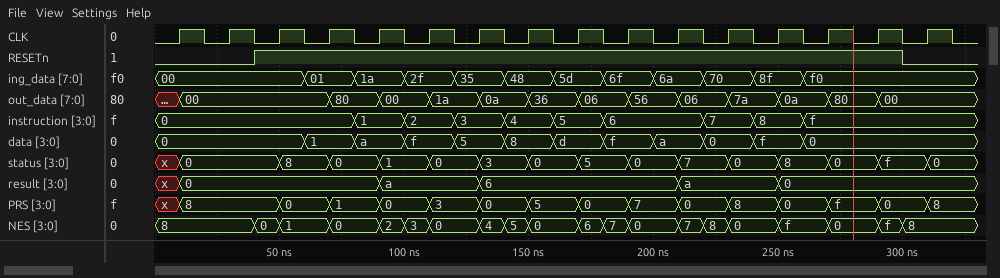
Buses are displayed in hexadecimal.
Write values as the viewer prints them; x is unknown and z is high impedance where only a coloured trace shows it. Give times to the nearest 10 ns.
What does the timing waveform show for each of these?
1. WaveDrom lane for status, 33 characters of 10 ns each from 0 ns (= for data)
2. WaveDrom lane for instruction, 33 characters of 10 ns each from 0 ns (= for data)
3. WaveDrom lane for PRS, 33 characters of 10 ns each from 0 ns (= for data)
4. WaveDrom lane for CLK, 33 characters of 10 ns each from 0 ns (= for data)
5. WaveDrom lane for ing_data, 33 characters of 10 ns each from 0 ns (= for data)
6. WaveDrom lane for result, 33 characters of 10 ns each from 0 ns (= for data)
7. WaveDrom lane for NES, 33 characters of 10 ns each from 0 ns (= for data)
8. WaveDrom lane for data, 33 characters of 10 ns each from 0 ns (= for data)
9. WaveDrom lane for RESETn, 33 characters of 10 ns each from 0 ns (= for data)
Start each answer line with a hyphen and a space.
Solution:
- {name: 'status', wave: 'x=...=.=.=.=.=.=.=.=.=.=.=.=.=.=.', data: '0 8 0 1 0 3 0 5 0 7 0 8 0 f 0'}
- {name: 'instruction', wave: '=.......=.=.=.=.=.=...=.=.=......', data: '0 1 2 3 4 5 6 7 8 f'}
- {name: 'PRS', wave: 'x=...=.=.=.=.=.=.=.=.=.=.=.=.=.=.', data: '8 0 1 0 3 0 5 0 7 0 8 0 f 0 8'}
- {name: 'CLK', wave: '010101010101010101010101010101010'}
- {name: 'ing_data', wave: '=.....=.=.=.=.=.=.=.=.=.=.=......', data: '00 01 1a 2f 35 48 5d 6f 6a 70 8f f0'}
- {name: 'result', wave: 'x=.......=...=.......=...=.......', data: '0 a 6 a 0'}
- {name: 'NES', wave: '=...==.=.===.===.===.===.=.=.==..', data: '8 0 1 0 2 3 0 4 5 0 6 7 0 7 8 0 f 0 f 8'}
- {name: 'data', wave: '=.....=.=.=.=.=.=.=.=.=.=.=......', data: '0 1 a f 5 8 d f a 0 f 0'}
- {name: 'RESETn', wave: '0...1.........................0..'}
